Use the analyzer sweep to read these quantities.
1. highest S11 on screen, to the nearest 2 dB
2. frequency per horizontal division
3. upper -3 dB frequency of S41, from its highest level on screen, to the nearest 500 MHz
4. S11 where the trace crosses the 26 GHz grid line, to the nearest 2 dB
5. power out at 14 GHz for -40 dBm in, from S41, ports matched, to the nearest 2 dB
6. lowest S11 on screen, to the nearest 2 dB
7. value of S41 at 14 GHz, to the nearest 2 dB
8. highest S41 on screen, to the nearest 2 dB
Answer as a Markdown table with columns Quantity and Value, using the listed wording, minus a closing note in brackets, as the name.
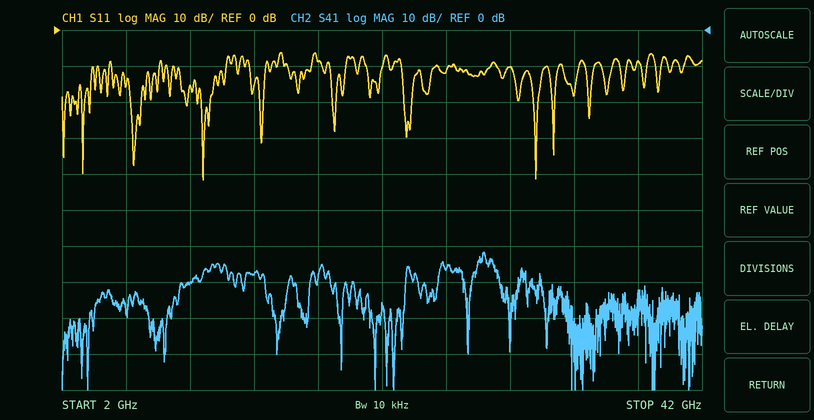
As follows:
| Quantity | Value |
|---|---|
| highest S11 on screen, to the nearest 2 dB | -6 dB |
| frequency per horizontal division | 4 GHz |
| upper -3 dB frequency of S41, from its highest level on screen, to the nearest 500 MHz | 28.5 GHz |
| S11 where the trace crosses the 26 GHz grid line, to the nearest 2 dB | -12 dB |
| power out at 14 GHz for -40 dBm in, from S41, ports matched, to the nearest 2 dB | -108 dBm |
| lowest S11 on screen, to the nearest 2 dB | -42 dB |
| value of S41 at 14 GHz, to the nearest 2 dB | -68 dB |
| highest S41 on screen, to the nearest 2 dB | -62 dB |
